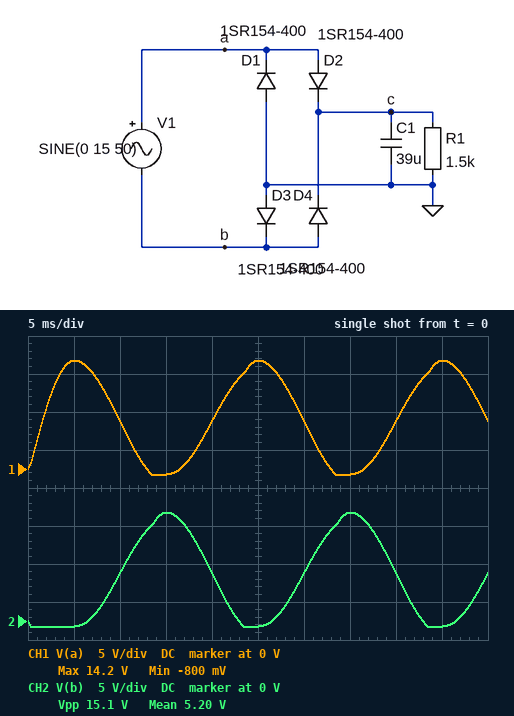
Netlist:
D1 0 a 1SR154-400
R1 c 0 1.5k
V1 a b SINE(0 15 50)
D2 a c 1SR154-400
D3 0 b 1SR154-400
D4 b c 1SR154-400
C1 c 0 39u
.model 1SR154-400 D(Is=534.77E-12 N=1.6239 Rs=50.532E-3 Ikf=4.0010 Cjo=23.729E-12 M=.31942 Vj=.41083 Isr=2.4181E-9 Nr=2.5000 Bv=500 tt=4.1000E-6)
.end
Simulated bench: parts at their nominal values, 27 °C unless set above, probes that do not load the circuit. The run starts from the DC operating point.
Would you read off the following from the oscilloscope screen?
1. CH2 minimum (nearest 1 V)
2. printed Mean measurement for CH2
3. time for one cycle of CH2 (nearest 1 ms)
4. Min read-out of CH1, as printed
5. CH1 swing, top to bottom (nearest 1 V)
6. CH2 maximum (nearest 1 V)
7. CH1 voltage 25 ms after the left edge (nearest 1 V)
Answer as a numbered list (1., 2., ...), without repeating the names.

1. -1 V
2. 5.20 V
3. 20 ms
4. -800 mV
5. 15 V
6. 14 V
7. 14 V
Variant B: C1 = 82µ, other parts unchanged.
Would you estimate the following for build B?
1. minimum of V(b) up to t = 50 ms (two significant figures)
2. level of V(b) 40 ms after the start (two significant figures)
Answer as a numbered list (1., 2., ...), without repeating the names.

1. -890 mV
2. 6.5 V
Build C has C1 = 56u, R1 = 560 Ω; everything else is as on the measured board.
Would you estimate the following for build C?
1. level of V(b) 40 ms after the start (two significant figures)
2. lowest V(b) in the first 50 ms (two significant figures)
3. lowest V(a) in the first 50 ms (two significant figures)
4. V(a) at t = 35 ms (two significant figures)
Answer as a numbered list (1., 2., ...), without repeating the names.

1. 5.8 V
2. -860 mV
3. -840 mV
4. -760 mV
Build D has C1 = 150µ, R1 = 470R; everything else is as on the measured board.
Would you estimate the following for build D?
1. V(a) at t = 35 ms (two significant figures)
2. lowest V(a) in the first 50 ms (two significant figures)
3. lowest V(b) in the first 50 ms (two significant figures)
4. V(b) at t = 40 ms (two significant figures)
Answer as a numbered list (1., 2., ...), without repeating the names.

1. -790 mV
2. -870 mV
3. -930 mV
4. 6.3 V
